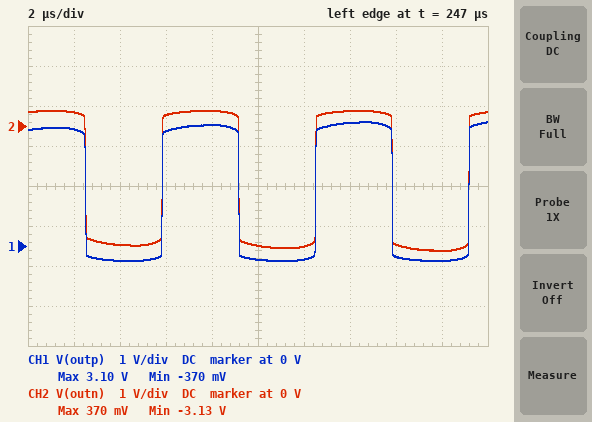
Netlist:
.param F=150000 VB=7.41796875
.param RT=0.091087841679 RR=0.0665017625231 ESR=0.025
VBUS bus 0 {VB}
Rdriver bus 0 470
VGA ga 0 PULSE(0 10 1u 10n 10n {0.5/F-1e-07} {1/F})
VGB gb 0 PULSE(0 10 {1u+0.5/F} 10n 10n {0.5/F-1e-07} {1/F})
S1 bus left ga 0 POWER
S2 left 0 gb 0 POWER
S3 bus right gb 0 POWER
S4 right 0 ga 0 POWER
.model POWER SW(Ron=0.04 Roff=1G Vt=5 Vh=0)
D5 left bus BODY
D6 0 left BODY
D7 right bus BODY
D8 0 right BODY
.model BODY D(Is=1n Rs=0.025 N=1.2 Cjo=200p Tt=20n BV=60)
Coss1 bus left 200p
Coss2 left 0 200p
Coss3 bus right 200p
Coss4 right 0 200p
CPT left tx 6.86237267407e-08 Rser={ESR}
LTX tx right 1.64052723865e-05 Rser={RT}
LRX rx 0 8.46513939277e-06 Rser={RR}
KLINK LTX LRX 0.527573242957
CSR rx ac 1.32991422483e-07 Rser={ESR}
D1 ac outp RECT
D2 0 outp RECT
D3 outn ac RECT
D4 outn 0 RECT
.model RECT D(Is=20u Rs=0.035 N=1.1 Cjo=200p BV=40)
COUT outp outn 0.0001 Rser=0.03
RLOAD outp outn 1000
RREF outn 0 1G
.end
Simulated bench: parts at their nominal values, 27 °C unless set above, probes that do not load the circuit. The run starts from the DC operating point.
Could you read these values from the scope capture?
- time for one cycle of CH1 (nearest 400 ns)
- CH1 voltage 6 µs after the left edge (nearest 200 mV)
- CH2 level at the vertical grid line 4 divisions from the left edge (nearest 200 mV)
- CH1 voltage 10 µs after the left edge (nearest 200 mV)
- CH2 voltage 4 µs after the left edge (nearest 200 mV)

6.8 µs
2.8 V
400 mV
-400 mV
-3.0 V
